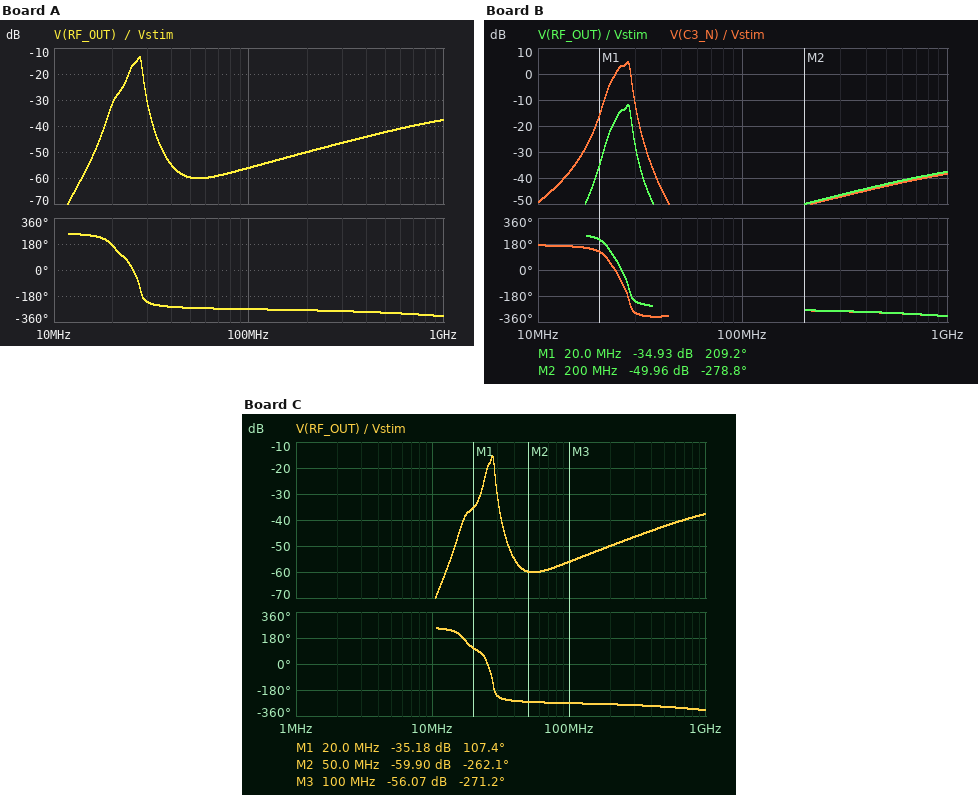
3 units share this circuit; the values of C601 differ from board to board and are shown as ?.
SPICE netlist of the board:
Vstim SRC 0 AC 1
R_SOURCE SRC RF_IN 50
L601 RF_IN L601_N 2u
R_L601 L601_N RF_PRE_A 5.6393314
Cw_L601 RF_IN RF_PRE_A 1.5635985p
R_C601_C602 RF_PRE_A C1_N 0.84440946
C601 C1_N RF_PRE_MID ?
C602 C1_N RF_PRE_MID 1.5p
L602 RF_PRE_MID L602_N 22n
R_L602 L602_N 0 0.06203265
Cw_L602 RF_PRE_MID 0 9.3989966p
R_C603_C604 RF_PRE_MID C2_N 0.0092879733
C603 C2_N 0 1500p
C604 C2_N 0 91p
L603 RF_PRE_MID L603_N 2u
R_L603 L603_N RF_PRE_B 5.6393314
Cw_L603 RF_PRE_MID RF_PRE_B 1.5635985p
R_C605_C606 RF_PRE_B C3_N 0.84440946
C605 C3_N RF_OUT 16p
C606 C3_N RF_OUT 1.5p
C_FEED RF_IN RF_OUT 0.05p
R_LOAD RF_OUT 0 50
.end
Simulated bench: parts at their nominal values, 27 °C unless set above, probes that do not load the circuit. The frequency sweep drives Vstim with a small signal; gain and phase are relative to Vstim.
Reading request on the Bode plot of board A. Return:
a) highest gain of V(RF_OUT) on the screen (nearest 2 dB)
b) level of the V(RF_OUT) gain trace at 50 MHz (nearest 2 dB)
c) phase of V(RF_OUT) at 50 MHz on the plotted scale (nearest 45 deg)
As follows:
-14 dB
-60 dB
-270 deg
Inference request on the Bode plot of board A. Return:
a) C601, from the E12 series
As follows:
27 pF
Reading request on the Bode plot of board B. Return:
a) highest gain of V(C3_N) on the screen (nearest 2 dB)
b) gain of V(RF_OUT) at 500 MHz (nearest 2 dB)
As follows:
4 dB
-42 dB
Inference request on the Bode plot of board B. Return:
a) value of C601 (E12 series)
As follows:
22 pF
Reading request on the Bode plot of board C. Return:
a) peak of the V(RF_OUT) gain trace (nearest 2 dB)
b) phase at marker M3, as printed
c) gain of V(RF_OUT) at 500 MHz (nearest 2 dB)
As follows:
-16 dB
-271.2 deg
-42 dB
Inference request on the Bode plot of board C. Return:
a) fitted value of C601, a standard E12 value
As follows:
39 pF
